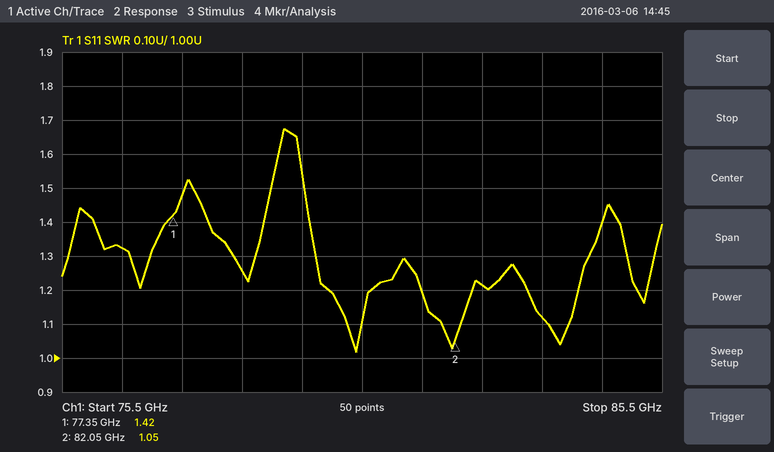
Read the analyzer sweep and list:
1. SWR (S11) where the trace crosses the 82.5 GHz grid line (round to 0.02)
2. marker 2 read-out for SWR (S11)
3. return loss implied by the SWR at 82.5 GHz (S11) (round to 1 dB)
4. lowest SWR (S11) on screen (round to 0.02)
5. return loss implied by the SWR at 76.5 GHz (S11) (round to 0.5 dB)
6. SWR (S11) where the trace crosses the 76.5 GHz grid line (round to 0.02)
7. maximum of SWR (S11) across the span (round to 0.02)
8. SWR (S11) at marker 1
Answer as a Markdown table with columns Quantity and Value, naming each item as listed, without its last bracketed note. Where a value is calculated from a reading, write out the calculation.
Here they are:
| Quantity | Value |
|---|---|
| SWR (S11) where the trace crosses the 82.5 GHz grid line | 1.22 |
| marker 2 read-out for SWR | 1.05 |
| return loss implied by the SWR at 82.5 GHz (S11) | −20 log10((1.22 − 1)/(1.22 + 1)) ≈ 20 dB |
| lowest SWR (S11) on screen | 1.02 |
| return loss implied by the SWR at 76.5 GHz (S11) | −20 log10((1.32 − 1)/(1.32 + 1)) ≈ 17.2 dB, so 17.0 dB to the nearest 0.5 dB |
| SWR (S11) where the trace crosses the 76.5 GHz grid line | 1.32 |
| maximum of SWR (S11) across the span | 1.68 |
| SWR (S11) at marker 1 | 1.42 |
